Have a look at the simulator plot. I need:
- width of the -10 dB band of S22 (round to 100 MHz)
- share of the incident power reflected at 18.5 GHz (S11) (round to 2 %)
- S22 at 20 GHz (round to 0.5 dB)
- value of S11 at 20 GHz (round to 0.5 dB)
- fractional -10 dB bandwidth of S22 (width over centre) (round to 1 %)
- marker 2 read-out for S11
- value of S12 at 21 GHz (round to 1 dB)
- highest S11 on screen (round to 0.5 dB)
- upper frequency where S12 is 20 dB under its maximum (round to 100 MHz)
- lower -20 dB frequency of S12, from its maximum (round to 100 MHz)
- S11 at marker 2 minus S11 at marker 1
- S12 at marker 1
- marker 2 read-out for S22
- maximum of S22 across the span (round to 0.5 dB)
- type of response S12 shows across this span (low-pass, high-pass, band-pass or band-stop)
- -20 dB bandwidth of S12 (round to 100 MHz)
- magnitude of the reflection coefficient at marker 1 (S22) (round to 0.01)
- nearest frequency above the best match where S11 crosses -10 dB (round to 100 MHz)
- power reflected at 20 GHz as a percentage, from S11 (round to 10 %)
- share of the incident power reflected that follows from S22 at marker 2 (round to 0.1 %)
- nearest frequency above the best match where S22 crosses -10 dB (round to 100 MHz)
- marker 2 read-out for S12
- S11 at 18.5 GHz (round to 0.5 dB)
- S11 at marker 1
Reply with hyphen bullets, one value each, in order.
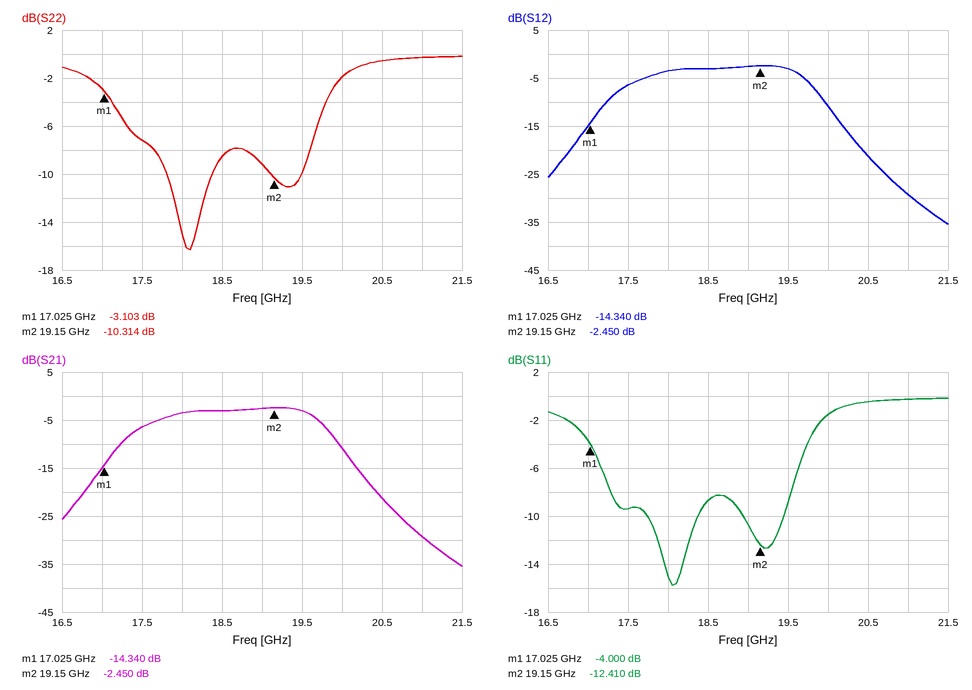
- 600 MHz
- 14 %
- -2.0 dB
- -1.5 dB
- 3 %
- -12.410 dB
- -29 dB
- 0.0 dB
- 20.6 GHz
- 16.7 GHz
- -8.410 dB
- -14.340 dB
- -10.314 dB
- 0.0 dB
- band-pass
- 3.9 GHz
- 0.70
- 18.4 GHz
- 70 %
- 9.3 %
- 18.4 GHz
- -2.450 dB
- -8.5 dB
- -4.000 dB
